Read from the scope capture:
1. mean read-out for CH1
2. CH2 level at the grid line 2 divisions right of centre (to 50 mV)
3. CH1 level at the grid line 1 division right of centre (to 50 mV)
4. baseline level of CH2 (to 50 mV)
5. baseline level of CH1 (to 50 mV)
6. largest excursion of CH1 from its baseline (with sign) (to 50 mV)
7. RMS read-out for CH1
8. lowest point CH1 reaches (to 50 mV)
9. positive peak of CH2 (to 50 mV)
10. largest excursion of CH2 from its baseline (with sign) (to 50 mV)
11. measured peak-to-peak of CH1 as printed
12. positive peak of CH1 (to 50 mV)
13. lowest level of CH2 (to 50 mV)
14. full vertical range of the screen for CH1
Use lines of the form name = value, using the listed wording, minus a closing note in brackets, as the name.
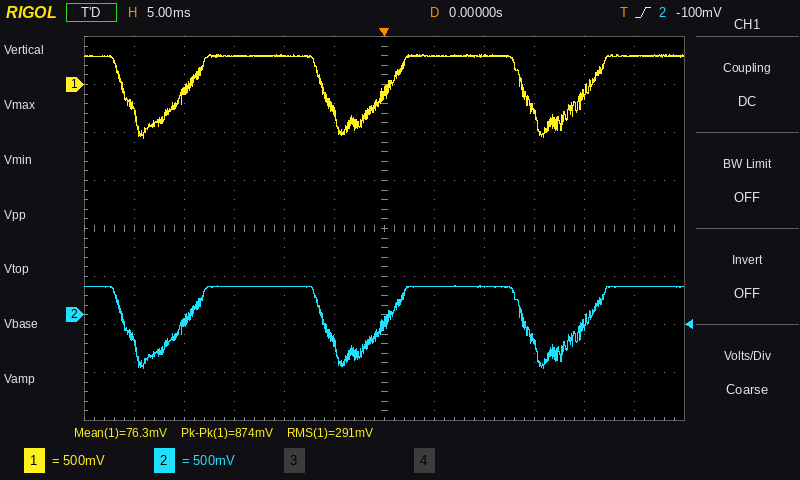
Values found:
mean read-out for CH1 = 76.3 mV
CH2 level at the grid line 2 divisions right of centre = 300 mV
CH1 level at the grid line 1 division right of centre = 300 mV
baseline level of CH2 = 300 mV
baseline level of CH1 = 300 mV
largest excursion of CH1 from its baseline (with sign) = -850 mV
RMS read-out for CH1 = 291 mV
lowest point CH1 reaches = -550 mV
positive peak of CH2 = 300 mV
largest excursion of CH2 from its baseline (with sign) = -850 mV
measured peak-to-peak of CH1 as printed = 874 mV
positive peak of CH1 = 300 mV
lowest level of CH2 = -550 mV
full vertical range of the screen for CH1 = 4 V
